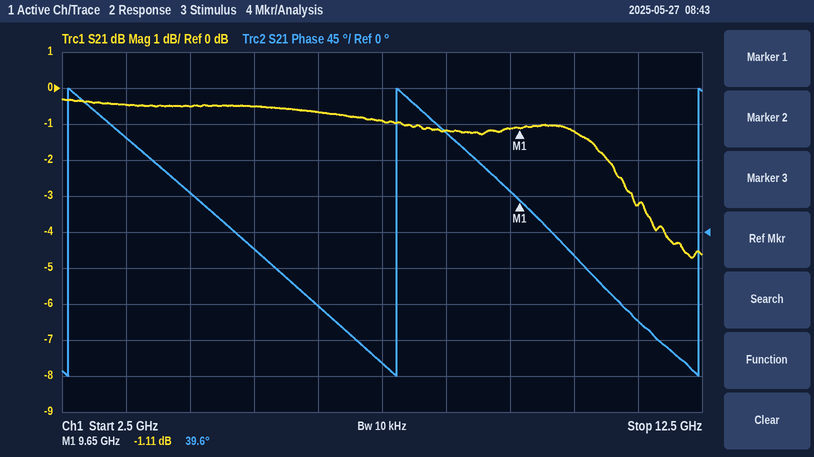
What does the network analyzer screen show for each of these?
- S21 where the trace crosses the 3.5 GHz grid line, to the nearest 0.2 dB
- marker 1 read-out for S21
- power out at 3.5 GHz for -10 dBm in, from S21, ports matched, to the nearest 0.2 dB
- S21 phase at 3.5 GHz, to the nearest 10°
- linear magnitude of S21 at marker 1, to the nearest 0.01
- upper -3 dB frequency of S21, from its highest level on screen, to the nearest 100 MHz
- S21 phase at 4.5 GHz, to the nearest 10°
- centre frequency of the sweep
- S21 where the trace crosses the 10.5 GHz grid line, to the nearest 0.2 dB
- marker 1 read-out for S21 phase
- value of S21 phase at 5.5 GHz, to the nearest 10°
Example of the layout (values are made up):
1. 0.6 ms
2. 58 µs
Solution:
1. -0.4 dB
2. -1.11 dB
3. -10.4 dBm
4. 120°
5. 0.88
6. 11.6 GHz
7. 50°
8. 7.5 GHz
9. -1.2 dB
10. 39.6°
11. -20°
